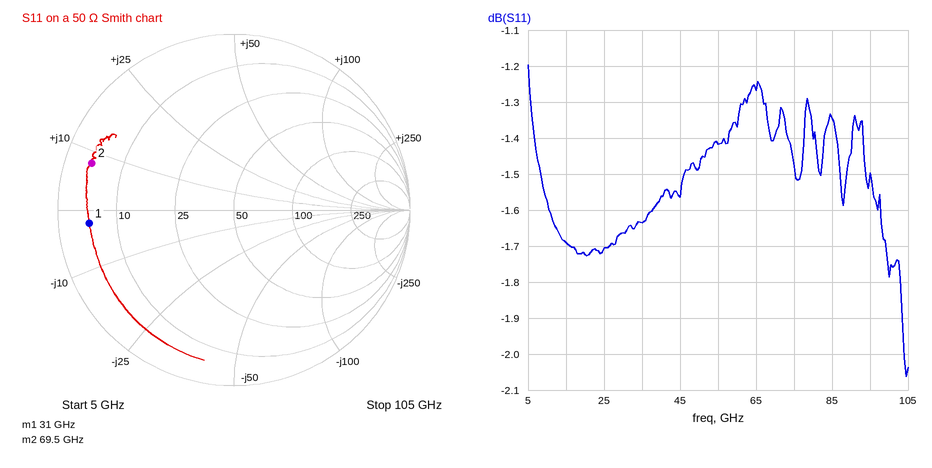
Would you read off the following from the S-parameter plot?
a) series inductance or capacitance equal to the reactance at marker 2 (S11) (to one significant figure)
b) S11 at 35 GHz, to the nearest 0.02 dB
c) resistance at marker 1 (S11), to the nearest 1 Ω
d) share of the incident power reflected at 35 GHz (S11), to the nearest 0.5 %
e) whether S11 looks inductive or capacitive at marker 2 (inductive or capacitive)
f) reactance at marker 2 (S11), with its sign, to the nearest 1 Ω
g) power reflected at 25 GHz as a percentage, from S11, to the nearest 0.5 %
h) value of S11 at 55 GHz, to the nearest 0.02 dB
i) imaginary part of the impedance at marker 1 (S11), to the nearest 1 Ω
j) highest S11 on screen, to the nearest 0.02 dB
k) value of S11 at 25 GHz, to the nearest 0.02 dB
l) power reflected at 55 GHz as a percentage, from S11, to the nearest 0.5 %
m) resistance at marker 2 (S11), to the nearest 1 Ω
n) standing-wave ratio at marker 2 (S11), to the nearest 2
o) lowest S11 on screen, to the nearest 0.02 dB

20 pH
-1.64 dB
5 Ω
68.5 %
inductive
+8 Ω
67.5 %
-1.42 dB
-2 Ω
-1.20 dB
-1.70 dB
72.0 %
4 Ω
12
-2.06 dB
